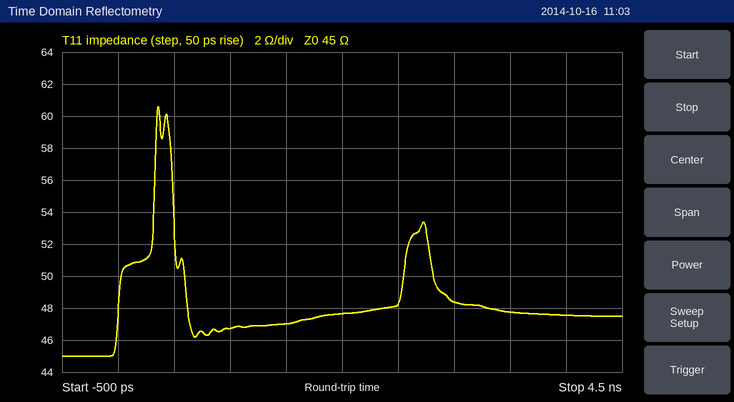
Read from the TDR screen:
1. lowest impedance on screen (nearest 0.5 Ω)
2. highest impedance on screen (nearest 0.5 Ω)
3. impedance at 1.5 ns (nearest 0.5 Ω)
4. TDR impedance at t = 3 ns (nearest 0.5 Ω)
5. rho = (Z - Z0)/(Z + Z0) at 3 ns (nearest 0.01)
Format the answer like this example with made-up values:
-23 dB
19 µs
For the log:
45.0 Ω
60.5 Ω
47.0 Ω
48.5 Ω
+0.04
